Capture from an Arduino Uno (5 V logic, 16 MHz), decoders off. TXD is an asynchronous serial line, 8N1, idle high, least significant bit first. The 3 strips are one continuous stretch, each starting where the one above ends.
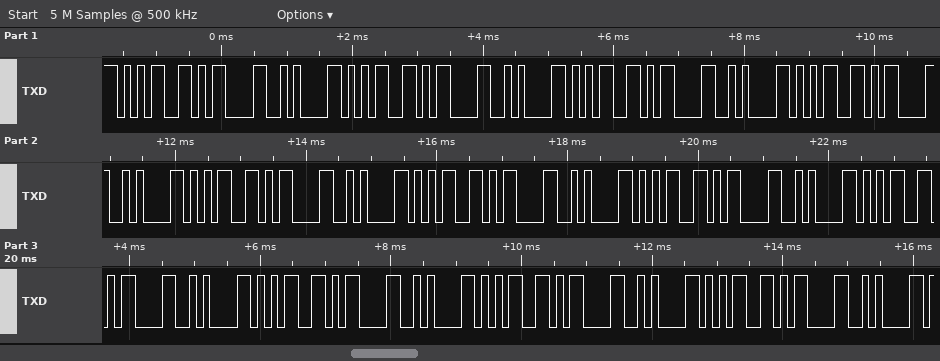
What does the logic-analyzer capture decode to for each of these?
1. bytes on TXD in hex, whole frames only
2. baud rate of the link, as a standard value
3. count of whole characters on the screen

35 0D 0A 35 0D 0A 35 0D 0A 35 0D 0A 35 0D 0A 35 0D 0A 35 0D 0A 35 0D 0A 35 0D 0A 35 0D 0A 35 0D 0A
9600 baud
33
